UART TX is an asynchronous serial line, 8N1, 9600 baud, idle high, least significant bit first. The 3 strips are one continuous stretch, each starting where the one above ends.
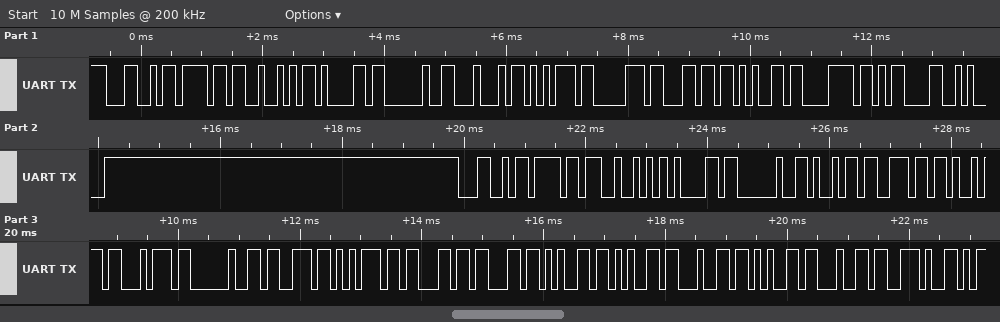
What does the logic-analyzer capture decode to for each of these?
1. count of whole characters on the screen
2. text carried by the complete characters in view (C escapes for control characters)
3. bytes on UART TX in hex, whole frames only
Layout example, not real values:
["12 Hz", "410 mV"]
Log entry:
["33", "\"LoRa Duplex\\r\\nLoRa init succeeded.\"", "0x4C 0x6F 0x52 0x61 0x20 0x44 0x75 0x70 0x6C 0x65 0x78 0x0D 0x0A 0x4C 0x6F 0x52 0x61 0x20 0x69 0x6E 0x69 0x74 0x20 0x73 0x75 0x63 0x63 0x65 0x65 0x64 0x65 0x64 0x2E"]
